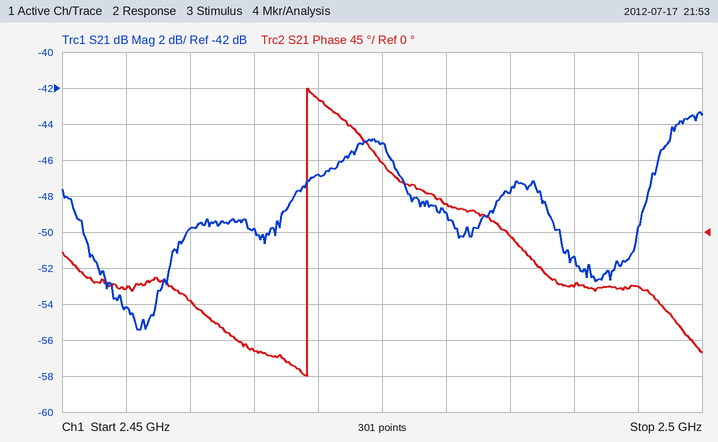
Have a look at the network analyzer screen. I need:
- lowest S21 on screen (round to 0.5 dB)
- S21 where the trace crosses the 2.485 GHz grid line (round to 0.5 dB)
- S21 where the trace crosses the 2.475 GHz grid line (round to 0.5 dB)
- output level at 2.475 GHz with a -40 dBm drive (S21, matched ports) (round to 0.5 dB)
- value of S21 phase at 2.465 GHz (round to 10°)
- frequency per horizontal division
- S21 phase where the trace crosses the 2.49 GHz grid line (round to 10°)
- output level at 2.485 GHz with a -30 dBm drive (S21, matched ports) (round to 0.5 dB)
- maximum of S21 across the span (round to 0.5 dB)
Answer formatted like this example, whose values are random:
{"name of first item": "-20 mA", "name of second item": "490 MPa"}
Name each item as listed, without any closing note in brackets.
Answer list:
{"lowest S21 on screen": "-55.5 dB", "S21 where the trace crosses the 2.485 GHz grid line": "-48.0 dB", "S21 where the trace crosses the 2.475 GHz grid line": "-45.0 dB", "output level at 2.475 GHz with a -40 dBm drive (S21, matched ports)": "-85.0 dBm", "value of S21 phase at 2.465 GHz": "-150°", "frequency per horizontal division": "5 MHz", "S21 phase where the trace crosses the 2.49 GHz grid line": "-70°", "output level at 2.485 GHz with a -30 dBm drive (S21, matched ports)": "-78.0 dBm", "maximum of S21 across the span": "-43.5 dB"}
